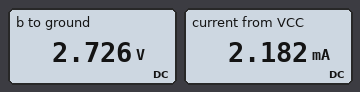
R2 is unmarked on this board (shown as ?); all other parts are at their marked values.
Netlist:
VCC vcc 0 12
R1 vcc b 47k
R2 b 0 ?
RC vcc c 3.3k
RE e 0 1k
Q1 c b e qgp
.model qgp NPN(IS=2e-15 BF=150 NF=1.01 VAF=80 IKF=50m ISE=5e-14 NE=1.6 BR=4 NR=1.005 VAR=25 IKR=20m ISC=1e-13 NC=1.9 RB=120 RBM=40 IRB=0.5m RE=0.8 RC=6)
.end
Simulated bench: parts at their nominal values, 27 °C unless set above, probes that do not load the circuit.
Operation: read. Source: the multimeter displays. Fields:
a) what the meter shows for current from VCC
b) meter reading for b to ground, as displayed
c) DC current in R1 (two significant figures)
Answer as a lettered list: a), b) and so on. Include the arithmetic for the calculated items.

a) 2.182 mA
b) 2.726 V
c) (12 V - 2.726 V) / 47 kΩ = 200 µA
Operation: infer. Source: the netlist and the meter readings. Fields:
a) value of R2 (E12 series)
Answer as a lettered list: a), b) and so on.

a) 15 kΩ
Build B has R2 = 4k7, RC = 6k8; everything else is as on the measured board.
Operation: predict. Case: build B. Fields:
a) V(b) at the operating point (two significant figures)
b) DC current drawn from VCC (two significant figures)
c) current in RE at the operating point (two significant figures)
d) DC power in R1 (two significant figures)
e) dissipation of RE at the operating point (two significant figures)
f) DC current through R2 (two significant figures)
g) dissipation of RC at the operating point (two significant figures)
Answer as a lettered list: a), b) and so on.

a) 1.1 V
b) 630 µA
c) 400 µA
d) 2.5 mW
e) 160 µW
f) 230 µA
g) 1.1 mW
